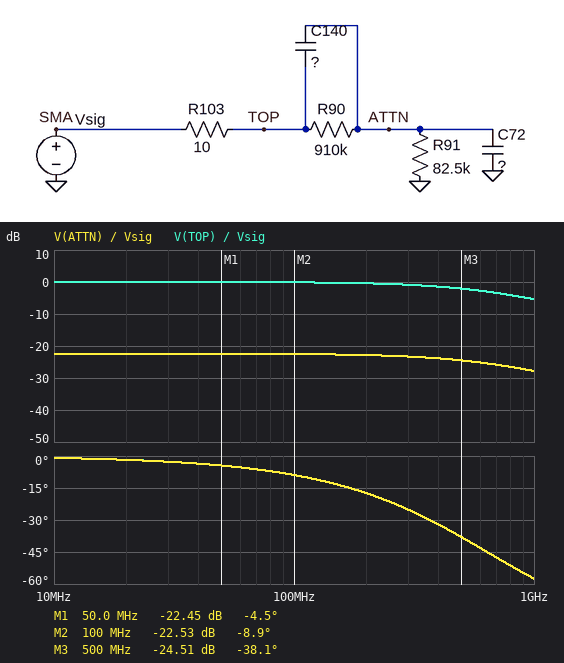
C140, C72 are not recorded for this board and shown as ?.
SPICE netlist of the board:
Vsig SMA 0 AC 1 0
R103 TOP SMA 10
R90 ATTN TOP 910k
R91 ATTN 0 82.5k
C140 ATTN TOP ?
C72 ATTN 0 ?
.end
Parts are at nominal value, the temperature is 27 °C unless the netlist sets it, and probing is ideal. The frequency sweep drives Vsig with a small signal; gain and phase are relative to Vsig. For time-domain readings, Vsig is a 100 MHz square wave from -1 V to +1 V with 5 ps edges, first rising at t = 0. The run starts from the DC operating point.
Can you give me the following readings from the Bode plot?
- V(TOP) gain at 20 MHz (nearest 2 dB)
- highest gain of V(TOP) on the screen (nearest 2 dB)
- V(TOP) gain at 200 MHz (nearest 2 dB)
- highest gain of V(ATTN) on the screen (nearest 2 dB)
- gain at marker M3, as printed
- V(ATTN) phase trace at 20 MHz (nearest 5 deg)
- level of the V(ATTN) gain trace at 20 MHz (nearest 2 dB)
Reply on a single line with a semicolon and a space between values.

0 dB; 0 dB; 0 dB; -22 dB; -24.51 dB; 0 deg; -22 dB
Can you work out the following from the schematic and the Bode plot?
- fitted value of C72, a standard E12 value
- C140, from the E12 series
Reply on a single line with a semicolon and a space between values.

330 pF; 27 pF
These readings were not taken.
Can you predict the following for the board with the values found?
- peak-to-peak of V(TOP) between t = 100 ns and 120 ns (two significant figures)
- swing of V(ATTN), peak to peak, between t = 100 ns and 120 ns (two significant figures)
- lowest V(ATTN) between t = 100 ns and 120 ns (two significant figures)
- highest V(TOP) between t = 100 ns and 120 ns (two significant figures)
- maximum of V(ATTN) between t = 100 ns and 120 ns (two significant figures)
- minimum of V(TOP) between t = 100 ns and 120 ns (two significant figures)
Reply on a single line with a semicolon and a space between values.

2.0 V; 150 mV; -83 mV; 1.0 V; 68 mV; -1.0 V
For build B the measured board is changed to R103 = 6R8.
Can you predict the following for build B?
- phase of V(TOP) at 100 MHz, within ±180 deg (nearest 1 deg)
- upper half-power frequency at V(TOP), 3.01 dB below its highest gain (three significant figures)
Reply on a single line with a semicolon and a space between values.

-6 deg; 938 MHz
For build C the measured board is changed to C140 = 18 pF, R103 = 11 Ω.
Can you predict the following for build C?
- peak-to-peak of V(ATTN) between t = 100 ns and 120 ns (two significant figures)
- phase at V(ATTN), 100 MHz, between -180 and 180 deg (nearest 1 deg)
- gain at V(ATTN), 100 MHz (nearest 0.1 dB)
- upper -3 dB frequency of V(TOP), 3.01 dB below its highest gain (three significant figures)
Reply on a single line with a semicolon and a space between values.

100 mV; -7 deg; -25.8 dB; 848 MHz
